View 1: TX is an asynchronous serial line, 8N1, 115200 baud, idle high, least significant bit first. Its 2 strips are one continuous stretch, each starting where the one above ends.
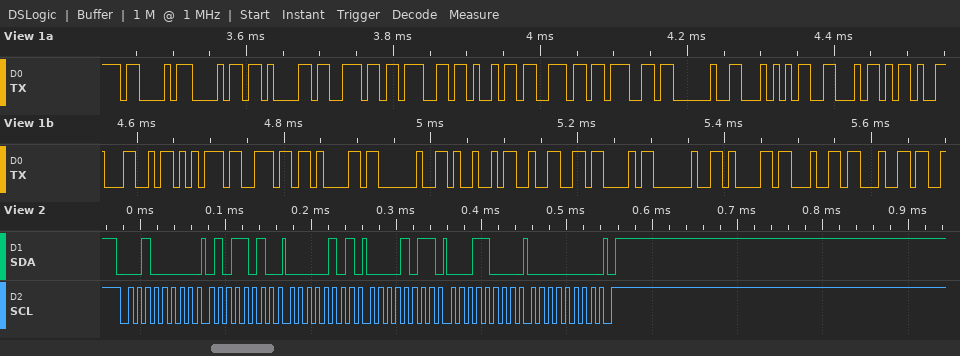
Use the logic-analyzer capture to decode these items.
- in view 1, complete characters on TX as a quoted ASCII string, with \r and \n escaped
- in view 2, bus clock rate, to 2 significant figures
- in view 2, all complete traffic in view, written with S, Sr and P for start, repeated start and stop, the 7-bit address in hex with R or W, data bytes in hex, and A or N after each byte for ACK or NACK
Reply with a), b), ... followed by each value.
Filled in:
a) "Changing TF-Luna I2C add"
b) 100 kHz
c) S 10W A 5A A 05 A 0B A 18 A 00 A P
